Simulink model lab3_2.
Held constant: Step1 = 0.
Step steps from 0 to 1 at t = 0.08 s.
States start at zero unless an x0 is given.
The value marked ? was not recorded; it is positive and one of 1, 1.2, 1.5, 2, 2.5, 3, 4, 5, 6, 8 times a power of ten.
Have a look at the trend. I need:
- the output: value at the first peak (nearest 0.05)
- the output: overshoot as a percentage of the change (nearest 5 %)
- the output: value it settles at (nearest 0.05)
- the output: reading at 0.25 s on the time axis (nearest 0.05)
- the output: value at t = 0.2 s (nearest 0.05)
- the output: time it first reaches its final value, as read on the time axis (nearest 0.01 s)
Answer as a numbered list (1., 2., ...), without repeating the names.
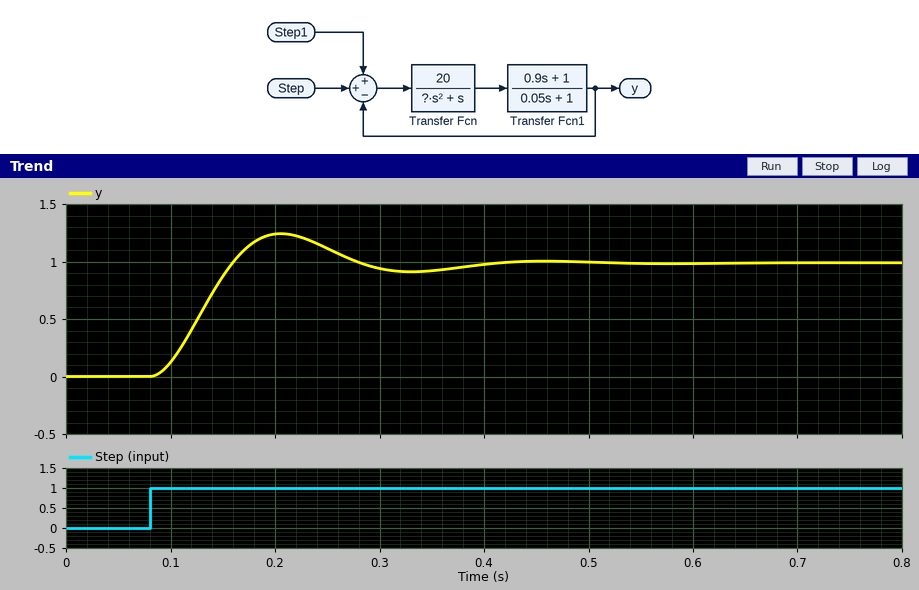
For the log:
1. 1.25
2. 25 %
3. 1.00
4. 1.10
5. 1.25
6. 0.16 s
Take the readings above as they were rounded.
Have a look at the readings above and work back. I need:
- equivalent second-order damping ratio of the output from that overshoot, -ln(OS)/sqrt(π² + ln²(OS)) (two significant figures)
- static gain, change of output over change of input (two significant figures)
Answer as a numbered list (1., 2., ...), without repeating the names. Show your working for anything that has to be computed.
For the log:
1. ln(0.25) = -1.386; 1.386 / sqrt(9.870 + 1.922) = 0.40
2. (1 - 0) / (1 - 0) = 1.0
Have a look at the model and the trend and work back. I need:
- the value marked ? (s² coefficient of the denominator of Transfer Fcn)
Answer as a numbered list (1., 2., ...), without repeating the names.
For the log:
1. 0.5
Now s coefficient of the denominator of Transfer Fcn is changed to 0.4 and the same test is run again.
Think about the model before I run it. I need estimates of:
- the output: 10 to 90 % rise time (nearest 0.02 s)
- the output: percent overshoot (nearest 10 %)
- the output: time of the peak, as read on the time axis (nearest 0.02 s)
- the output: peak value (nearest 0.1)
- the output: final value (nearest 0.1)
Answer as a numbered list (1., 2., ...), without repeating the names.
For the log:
1. 0.06 s
2. 30 %
3. 0.20 s
4. 1.3
5. 1.0
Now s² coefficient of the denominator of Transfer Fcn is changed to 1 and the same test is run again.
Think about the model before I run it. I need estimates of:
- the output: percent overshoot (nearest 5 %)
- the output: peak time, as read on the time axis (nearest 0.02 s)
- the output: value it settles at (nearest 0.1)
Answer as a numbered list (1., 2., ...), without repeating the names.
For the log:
1. 15 %
2. 0.28 s
3. 1.0
